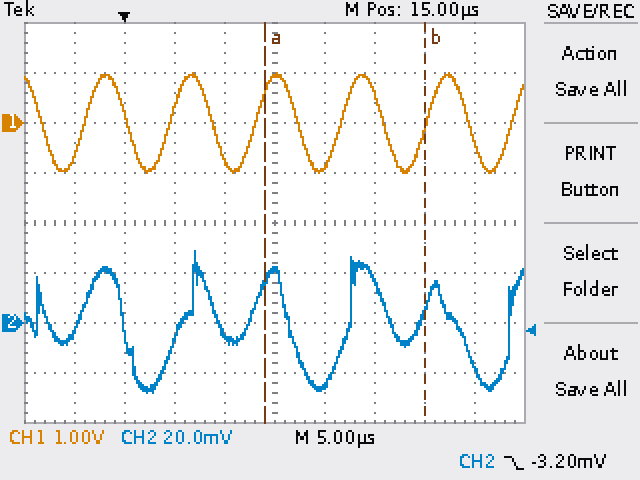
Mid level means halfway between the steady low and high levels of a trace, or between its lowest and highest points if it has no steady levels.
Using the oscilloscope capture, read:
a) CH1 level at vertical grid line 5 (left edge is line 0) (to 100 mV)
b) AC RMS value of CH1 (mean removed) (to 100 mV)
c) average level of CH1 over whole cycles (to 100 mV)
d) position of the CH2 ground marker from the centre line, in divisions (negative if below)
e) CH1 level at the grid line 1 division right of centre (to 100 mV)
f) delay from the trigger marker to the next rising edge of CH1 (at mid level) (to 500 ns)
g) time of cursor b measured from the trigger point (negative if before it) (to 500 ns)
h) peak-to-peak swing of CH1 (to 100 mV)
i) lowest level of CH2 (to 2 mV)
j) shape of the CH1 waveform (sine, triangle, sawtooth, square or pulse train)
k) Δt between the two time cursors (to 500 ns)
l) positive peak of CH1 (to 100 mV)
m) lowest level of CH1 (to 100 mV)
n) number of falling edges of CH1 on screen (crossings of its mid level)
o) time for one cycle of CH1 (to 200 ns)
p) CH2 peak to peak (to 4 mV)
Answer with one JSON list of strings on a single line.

["900 mV", "700 mV", "0.0 V", "-2.0 div", "-900 mV", "4.5 µs", "+30.0 µs", "2.0 V", "-28 mV", "sine", "16.0 µs", "1.0 V", "-1.0 V", "6", "8.6 µs", "56 mV"]
